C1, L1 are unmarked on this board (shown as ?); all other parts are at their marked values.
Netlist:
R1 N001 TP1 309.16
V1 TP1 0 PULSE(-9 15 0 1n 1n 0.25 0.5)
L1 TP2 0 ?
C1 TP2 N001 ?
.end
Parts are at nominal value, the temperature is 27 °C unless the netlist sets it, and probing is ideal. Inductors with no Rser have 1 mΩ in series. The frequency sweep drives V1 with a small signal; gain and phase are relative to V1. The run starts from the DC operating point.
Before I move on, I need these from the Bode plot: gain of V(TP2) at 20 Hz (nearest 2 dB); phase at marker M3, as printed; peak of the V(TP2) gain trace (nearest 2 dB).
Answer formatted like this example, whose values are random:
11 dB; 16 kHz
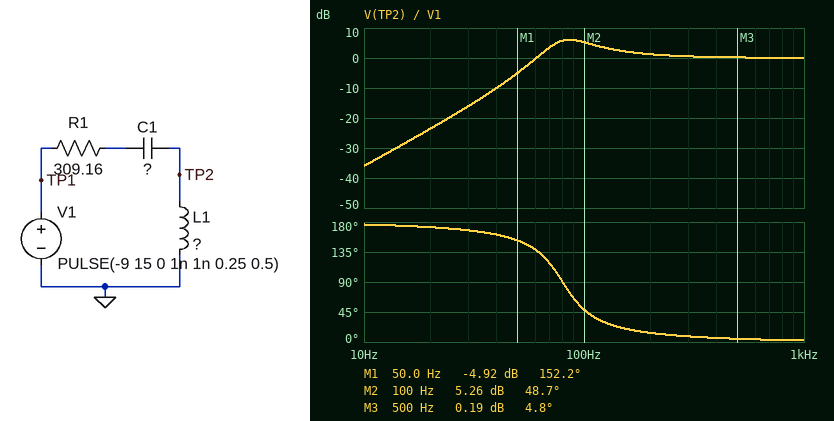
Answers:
-24 dB; 4.8 deg; 6 dB
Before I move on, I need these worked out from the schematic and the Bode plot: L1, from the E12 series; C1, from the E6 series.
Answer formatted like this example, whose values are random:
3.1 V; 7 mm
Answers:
1.2 H; 3.3 µF
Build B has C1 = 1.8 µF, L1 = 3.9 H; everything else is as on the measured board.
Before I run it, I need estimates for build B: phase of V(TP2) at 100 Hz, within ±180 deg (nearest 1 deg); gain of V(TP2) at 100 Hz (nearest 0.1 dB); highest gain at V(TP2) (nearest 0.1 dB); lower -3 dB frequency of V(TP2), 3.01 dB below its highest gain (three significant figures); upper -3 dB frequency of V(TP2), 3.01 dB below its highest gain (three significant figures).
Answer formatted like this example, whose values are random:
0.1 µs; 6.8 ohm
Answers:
11 deg; 3.7 dB; 13.6 dB; 55.1 Hz; 68.5 Hz
